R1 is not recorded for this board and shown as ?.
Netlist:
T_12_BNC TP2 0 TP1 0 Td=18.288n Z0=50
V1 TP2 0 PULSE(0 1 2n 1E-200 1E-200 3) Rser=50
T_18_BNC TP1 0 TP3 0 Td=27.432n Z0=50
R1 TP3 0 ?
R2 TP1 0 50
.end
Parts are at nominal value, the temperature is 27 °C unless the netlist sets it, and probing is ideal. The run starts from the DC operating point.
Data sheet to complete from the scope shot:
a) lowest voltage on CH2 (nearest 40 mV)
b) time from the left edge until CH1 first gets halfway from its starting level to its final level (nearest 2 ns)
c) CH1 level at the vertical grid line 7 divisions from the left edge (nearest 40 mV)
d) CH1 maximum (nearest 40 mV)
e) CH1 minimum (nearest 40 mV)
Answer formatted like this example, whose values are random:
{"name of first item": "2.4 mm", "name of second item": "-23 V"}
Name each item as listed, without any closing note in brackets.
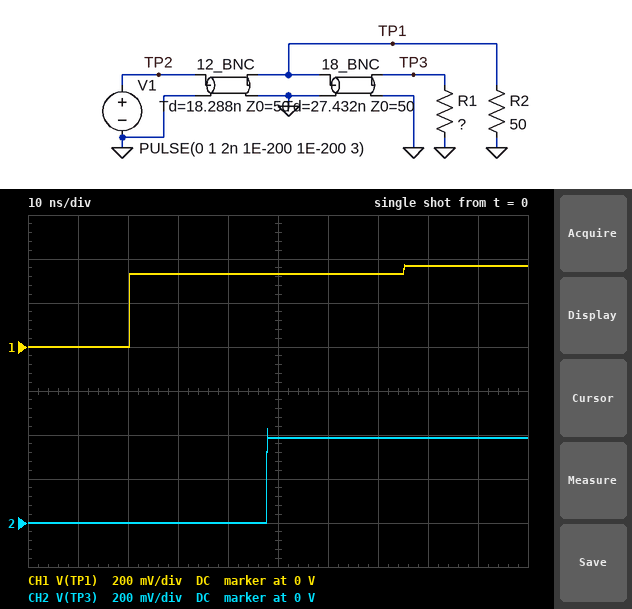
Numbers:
{"lowest voltage on CH2": "0 V", "time from the left edge until CH1 first gets halfway from its starting level to its final level": "20 ns", "CH1 level at the vertical grid line 7 divisions from the left edge": "320 mV", "CH1 maximum": "360 mV", "CH1 minimum": "0 V"}
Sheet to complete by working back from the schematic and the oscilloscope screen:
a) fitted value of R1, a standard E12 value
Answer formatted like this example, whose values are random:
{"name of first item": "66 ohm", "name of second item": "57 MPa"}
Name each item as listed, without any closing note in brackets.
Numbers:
{"fitted value of R1, a standard E12 value": "68 Ω"}
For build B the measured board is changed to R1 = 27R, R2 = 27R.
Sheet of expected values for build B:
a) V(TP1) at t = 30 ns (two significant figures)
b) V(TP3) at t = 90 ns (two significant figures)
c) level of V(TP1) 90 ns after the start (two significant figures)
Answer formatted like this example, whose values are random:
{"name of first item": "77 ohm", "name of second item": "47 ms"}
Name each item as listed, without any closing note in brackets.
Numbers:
{"V(TP1) at t = 30 ns": "260 mV", "V(TP3) at t = 90 ns": "180 mV", "level of V(TP1) 90 ns after the start": "220 mV"}
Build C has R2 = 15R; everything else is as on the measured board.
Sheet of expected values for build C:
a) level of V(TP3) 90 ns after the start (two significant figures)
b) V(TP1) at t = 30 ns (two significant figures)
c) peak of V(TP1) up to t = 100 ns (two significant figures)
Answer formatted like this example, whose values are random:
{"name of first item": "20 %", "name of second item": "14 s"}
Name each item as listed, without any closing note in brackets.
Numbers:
{"level of V(TP3) 90 ns after the start": "220 mV", "V(TP1) at t = 30 ns": "190 mV", "peak of V(TP1) up to t = 100 ns": "200 mV"}
